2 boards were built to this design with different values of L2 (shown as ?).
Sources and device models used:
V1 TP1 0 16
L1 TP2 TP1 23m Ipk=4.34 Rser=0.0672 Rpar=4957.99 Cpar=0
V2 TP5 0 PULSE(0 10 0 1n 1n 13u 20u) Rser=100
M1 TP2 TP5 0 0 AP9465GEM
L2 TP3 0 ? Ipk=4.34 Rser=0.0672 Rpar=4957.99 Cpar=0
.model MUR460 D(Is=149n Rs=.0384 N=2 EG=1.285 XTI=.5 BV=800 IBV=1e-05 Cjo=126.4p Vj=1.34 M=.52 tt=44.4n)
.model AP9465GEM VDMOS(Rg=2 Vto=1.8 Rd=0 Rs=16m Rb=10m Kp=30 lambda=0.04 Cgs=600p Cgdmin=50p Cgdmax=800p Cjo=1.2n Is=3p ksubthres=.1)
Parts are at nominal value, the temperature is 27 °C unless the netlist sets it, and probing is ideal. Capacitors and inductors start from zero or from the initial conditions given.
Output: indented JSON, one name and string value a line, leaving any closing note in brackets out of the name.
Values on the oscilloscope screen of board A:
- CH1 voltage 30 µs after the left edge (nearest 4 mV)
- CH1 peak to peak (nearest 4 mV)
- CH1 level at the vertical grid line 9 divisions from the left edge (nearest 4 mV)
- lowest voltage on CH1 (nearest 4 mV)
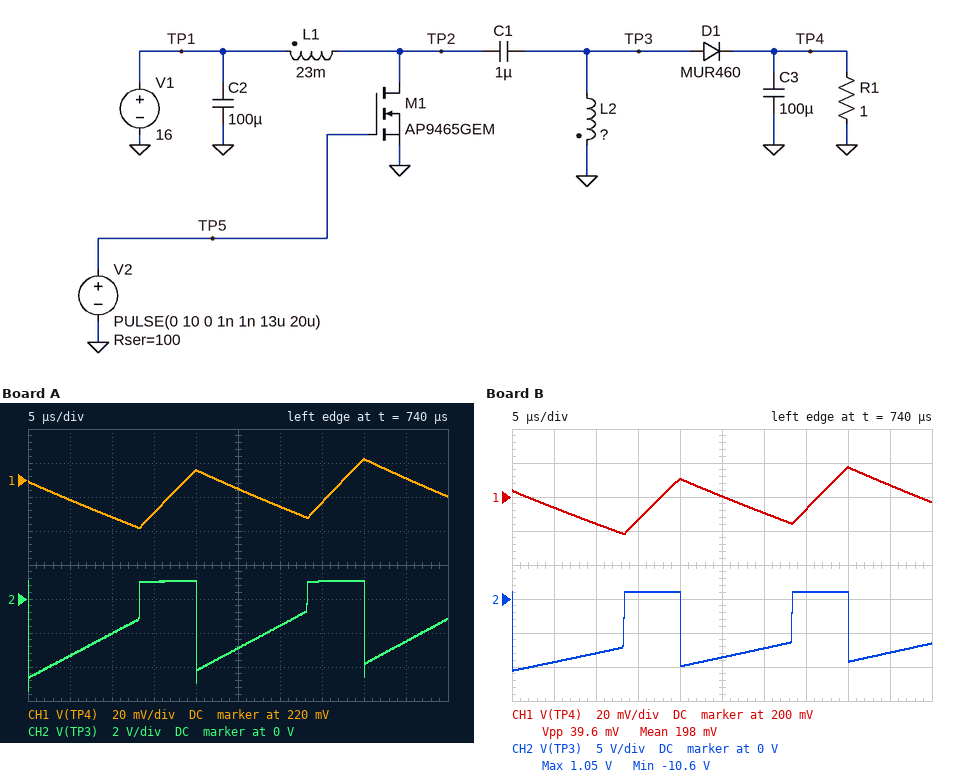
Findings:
{
  "CH1 voltage 30 µs after the left edge": "204 mV",
  "CH1 peak to peak": "40 mV",
  "CH1 level at the vertical grid line 9 divisions from the left edge": "220 mV",
  "lowest voltage on CH1": "192 mV"
}
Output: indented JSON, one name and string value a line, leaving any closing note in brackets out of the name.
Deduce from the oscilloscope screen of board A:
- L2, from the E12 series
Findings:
{
  "L2, from the E12 series": "10 mH"
}
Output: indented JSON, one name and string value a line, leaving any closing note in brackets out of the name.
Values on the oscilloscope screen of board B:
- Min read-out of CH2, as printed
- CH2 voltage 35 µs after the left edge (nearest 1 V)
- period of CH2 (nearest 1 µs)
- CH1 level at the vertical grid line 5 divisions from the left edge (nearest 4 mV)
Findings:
{
  "Min read-out of CH2, as printed": "-10.6 V",
  "CH2 voltage 35 µs after the left edge": "1 V",
  "period of CH2": "20 µs",
  "CH1 level at the vertical grid line 5 divisions from the left edge": "200 mV"
}
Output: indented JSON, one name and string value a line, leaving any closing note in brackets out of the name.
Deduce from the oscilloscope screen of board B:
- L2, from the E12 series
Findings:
{
  "L2, from the E12 series": "15 mH"
}
